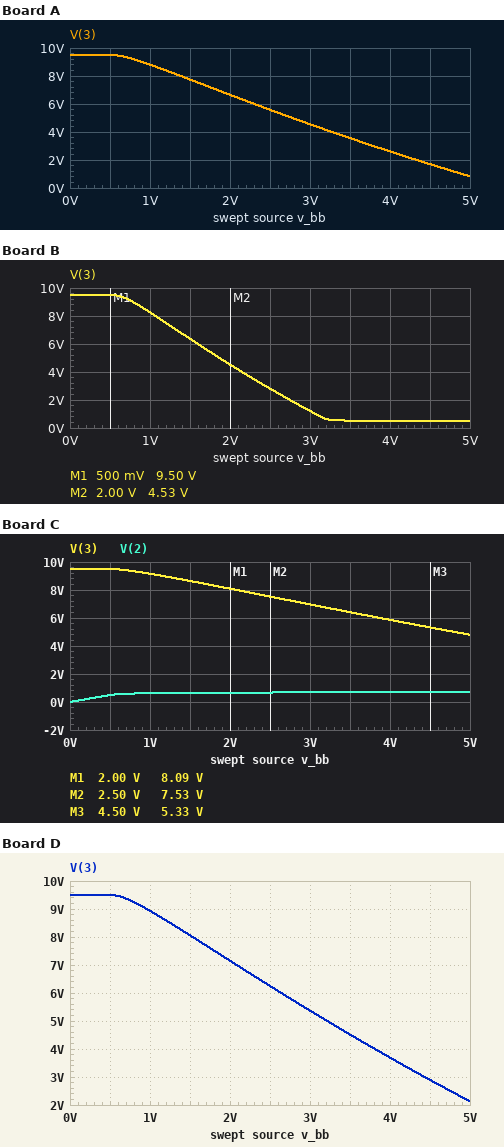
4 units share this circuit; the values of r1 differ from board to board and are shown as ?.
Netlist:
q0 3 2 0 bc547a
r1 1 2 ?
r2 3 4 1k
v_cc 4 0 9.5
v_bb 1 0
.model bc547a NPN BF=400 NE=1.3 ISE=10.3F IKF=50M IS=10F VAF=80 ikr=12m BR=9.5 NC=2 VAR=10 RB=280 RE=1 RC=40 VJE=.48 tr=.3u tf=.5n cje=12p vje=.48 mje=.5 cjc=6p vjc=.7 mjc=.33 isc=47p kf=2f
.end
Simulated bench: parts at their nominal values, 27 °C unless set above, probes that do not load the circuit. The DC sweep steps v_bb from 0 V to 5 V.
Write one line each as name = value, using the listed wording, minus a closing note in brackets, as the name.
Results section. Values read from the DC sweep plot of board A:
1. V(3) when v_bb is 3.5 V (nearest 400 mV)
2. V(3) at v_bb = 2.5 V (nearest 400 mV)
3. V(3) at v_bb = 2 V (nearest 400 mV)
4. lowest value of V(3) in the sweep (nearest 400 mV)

V(3) when v_bb is 3.5 V = 3.6 V
V(3) at v_bb = 2.5 V = 5.6 V
V(3) at v_bb = 2 V = 6.8 V
lowest value of V(3) in the sweep = 800 mV
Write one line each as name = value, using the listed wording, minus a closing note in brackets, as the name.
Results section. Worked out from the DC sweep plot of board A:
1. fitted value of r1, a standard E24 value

fitted value of r1, a standard E24 value = 91 kΩ
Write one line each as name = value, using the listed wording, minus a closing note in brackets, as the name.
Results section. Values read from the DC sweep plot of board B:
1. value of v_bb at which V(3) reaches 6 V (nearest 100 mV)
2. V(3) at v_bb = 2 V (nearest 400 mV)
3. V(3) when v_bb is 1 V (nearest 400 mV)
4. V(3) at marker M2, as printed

value of v_bb at which V(3) reaches 6 V = 1.6 V
V(3) at v_bb = 2 V = 4.4 V
V(3) when v_bb is 1 V = 8.4 V
V(3) at marker M2, as printed = 4.53 V
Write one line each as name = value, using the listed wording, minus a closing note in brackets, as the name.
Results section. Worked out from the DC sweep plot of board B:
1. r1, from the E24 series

r1, from the E24 series = 51 kΩ
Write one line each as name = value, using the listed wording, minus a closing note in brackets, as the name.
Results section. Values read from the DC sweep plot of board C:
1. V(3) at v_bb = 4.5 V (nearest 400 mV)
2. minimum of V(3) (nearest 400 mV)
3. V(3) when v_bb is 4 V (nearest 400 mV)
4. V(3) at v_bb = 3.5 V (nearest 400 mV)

V(3) at v_bb = 4.5 V = 5.2 V
minimum of V(3) = 4.8 V
V(3) when v_bb is 4 V = 6.0 V
V(3) at v_bb = 3.5 V = 6.4 V
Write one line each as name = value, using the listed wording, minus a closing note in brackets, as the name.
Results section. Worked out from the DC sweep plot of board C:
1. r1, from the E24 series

r1, from the E24 series = 180 kΩ
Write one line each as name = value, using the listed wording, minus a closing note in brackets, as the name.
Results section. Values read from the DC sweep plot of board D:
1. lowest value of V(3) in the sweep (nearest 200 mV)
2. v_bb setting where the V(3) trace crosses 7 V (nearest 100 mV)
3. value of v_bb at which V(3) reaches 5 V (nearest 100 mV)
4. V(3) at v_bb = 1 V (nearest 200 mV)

lowest value of V(3) in the sweep = 2.2 V
v_bb setting where the V(3) trace crosses 7 V = 2.1 V
value of v_bb at which V(3) reaches 5 V = 3.2 V
V(3) at v_bb = 1 V = 9.0 V
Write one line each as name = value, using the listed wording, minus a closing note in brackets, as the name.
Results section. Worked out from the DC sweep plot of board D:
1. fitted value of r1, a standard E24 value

fitted value of r1, a standard E24 value = 110 kΩ
